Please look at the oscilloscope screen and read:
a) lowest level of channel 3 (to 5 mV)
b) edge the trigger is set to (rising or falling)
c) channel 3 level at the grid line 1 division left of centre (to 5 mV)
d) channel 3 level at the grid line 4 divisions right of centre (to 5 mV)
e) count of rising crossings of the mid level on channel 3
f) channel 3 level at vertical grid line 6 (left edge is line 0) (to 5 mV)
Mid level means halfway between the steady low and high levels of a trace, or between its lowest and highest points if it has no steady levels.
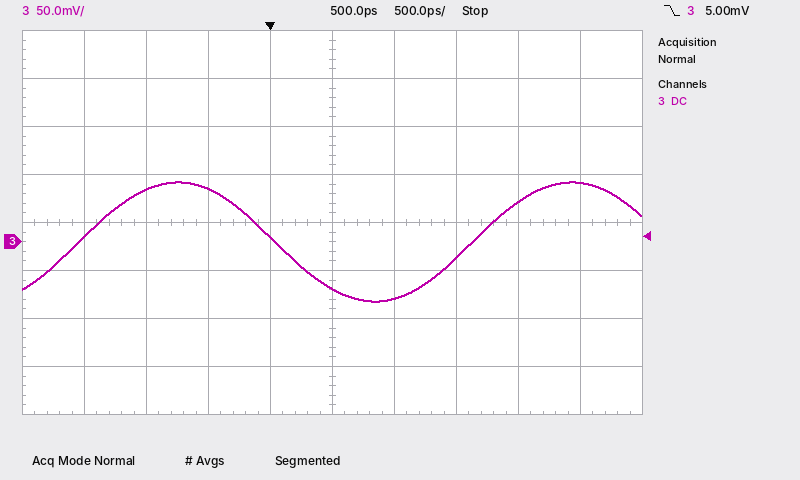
-60 mV
falling
5 mV
60 mV
2
-60 mV
